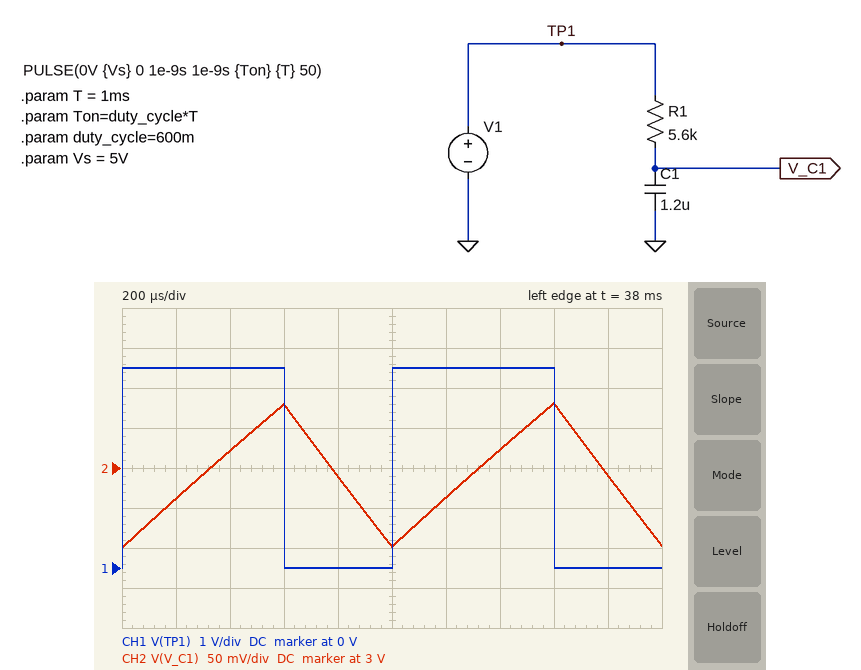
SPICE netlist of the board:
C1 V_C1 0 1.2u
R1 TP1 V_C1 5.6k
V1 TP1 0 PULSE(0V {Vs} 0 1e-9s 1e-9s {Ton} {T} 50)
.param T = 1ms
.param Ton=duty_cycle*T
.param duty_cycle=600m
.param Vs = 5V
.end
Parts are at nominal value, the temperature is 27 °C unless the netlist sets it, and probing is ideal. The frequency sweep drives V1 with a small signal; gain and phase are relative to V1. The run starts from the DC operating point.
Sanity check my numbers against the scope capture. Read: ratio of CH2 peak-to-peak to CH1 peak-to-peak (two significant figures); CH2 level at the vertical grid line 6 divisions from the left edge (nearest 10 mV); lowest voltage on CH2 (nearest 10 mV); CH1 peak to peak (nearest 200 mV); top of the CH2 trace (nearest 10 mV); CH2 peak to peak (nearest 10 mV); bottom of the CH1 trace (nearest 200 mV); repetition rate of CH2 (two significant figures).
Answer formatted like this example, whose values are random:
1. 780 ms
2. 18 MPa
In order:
1. 0.036
2. 2.96 V
3. 2.90 V
4. 5.0 V
5. 3.08 V
6. 180 mV
7. 0 V
8. 1.0 kHz
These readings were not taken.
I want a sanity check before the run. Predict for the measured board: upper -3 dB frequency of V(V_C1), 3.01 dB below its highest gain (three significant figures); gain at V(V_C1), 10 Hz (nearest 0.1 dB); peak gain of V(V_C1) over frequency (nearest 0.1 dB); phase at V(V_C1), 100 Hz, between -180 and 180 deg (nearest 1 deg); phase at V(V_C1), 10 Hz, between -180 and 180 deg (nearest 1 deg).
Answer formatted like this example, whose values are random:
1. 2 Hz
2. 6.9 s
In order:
1. 23.7 Hz
2. -0.7 dB
3. 0 dB
4. -77 deg
5. -23 deg
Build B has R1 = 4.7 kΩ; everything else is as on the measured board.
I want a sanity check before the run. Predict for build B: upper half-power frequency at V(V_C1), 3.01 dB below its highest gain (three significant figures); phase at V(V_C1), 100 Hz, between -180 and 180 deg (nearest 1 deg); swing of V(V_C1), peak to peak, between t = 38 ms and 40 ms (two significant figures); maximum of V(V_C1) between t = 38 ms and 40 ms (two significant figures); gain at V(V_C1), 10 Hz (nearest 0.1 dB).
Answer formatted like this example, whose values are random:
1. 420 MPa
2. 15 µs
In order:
1. 28.2 Hz
2. -74 deg
3. 210 mV
4. 3.1 V
5. -0.5 dB
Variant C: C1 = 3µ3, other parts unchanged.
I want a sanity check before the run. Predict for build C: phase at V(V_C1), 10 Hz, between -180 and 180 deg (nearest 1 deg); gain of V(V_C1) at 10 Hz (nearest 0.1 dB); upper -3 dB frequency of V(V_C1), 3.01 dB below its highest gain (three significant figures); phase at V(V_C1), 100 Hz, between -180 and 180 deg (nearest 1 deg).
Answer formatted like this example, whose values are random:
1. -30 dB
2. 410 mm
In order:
1. -49 deg
2. -3.7 dB
3. 8.61 Hz
4. -85 deg
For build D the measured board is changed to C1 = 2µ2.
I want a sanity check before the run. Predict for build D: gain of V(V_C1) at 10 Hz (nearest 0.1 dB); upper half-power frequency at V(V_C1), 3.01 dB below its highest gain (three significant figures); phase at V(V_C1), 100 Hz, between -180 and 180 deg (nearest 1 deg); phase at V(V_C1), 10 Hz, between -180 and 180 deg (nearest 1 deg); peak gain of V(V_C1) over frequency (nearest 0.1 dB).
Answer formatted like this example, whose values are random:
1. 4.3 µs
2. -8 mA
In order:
1. -2.0 dB
2. 12.9 Hz
3. -83 deg
4. -38 deg
5. 0 dB
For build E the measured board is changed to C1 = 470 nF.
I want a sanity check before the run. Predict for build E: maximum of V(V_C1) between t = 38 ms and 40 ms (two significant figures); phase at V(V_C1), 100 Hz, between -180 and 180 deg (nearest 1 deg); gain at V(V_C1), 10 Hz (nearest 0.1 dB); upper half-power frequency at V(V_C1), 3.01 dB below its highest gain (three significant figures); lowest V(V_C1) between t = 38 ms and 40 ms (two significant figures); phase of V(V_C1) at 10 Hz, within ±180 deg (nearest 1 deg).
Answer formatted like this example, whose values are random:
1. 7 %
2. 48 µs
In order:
1. 3.2 V
2. -59 deg
3. -0.1 dB
4. 60.5 Hz
5. 2.8 V
6. -9 deg
